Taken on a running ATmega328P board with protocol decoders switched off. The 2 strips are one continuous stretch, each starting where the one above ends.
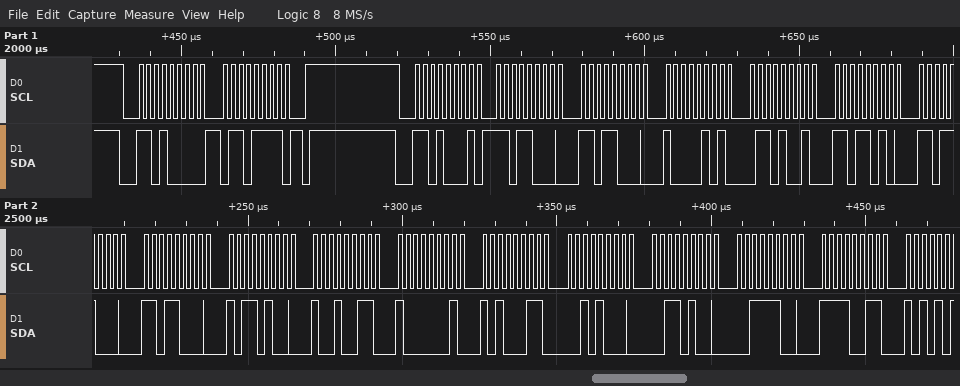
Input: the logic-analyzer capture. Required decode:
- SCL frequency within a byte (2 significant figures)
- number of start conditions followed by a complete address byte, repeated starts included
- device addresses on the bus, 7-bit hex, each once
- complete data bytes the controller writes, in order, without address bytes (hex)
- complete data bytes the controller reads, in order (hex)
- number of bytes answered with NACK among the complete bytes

400 kHz
2
0x68
6F
D8 D8 85 69 DA D8 D8 B4 93 81 A3 28 34 3C F3
0
